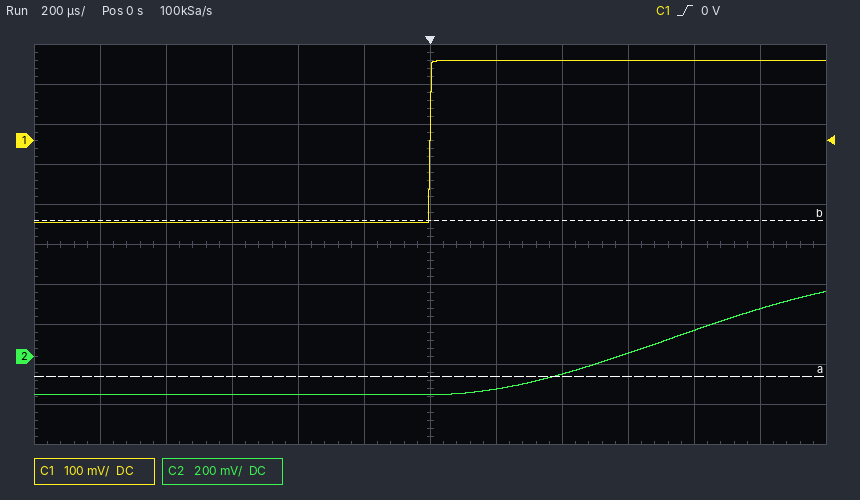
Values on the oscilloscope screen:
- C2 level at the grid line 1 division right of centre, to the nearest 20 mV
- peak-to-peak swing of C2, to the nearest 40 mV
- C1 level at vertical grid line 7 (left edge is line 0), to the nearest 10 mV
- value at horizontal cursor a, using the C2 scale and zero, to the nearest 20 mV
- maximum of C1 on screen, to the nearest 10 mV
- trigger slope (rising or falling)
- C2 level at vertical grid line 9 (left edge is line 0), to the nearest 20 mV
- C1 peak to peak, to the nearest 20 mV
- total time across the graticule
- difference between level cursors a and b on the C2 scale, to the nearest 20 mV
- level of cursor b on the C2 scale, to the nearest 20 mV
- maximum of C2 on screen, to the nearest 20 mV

-160 mV
520 mV
200 mV
-100 mV
200 mV
rising
20 mV
400 mV
2.4 ms
780 mV
680 mV
320 mV
